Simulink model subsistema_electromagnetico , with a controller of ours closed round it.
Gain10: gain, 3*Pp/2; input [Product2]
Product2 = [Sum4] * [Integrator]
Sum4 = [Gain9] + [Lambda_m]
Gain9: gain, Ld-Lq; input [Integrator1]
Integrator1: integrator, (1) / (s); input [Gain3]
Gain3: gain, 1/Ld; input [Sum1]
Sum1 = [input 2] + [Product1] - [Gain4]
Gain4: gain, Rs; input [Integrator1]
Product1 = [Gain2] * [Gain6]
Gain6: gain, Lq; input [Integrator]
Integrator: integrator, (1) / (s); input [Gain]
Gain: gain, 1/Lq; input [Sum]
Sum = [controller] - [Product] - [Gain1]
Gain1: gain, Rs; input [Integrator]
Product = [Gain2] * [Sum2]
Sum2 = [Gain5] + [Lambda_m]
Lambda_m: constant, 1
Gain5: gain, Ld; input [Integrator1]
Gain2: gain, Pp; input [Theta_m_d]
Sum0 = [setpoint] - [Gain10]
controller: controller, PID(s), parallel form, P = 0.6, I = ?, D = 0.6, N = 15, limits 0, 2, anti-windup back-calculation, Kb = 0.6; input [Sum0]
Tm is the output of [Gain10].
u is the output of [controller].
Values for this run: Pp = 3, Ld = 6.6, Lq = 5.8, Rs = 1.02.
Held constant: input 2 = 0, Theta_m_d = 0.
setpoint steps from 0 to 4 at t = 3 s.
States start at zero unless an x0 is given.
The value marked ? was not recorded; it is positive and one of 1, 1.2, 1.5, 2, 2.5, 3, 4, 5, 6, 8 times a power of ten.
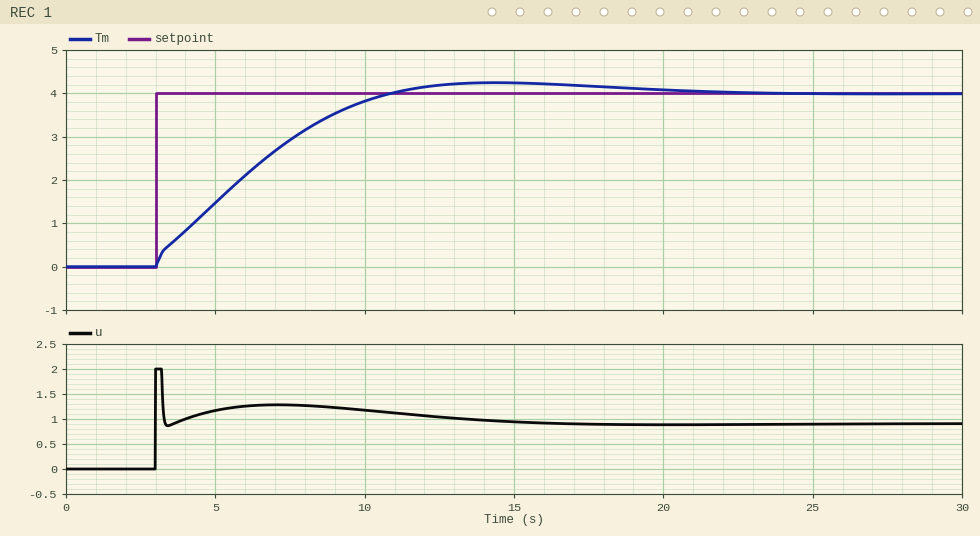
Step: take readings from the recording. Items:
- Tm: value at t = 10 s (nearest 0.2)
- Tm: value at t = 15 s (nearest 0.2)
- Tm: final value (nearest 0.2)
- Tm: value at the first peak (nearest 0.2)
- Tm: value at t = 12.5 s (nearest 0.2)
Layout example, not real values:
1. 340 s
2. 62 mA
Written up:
1. 3.8
2. 4.2
3. 4.0
4. 4.2
5. 4.2
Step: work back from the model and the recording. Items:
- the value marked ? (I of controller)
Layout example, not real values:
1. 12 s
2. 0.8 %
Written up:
1. 0.2
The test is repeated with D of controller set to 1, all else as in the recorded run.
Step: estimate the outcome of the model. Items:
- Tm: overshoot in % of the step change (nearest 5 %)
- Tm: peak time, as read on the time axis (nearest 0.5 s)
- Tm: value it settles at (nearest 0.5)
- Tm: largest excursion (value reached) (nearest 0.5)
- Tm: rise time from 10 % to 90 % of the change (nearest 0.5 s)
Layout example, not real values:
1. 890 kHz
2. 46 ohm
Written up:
1. 10 %
2. 16.5 s
3. 4.0
4. 4.5
5. 7.5 s
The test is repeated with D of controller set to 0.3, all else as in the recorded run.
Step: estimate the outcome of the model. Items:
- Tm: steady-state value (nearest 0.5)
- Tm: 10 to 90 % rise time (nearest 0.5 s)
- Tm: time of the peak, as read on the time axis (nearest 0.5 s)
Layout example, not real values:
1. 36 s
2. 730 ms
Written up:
1. 4.0
2. 4.5 s
3. 12.5 s
